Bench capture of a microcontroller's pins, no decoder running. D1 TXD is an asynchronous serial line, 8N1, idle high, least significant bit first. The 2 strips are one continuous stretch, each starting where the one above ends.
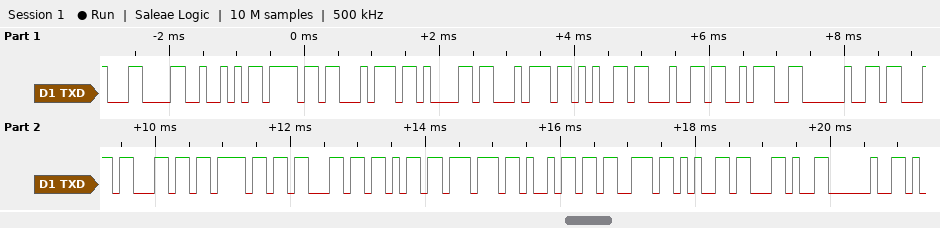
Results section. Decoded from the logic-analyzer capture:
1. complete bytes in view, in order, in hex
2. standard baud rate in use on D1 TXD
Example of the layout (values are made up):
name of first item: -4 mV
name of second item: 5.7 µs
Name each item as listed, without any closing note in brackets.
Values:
complete bytes in view, in order, in hex: 0C 52 6F 74 61 74 65 64 3A 20 63 6C 6F 63 6B 77 69 73 65 2C 20
standard baud rate in use on D1 TXD: 9600 baud
